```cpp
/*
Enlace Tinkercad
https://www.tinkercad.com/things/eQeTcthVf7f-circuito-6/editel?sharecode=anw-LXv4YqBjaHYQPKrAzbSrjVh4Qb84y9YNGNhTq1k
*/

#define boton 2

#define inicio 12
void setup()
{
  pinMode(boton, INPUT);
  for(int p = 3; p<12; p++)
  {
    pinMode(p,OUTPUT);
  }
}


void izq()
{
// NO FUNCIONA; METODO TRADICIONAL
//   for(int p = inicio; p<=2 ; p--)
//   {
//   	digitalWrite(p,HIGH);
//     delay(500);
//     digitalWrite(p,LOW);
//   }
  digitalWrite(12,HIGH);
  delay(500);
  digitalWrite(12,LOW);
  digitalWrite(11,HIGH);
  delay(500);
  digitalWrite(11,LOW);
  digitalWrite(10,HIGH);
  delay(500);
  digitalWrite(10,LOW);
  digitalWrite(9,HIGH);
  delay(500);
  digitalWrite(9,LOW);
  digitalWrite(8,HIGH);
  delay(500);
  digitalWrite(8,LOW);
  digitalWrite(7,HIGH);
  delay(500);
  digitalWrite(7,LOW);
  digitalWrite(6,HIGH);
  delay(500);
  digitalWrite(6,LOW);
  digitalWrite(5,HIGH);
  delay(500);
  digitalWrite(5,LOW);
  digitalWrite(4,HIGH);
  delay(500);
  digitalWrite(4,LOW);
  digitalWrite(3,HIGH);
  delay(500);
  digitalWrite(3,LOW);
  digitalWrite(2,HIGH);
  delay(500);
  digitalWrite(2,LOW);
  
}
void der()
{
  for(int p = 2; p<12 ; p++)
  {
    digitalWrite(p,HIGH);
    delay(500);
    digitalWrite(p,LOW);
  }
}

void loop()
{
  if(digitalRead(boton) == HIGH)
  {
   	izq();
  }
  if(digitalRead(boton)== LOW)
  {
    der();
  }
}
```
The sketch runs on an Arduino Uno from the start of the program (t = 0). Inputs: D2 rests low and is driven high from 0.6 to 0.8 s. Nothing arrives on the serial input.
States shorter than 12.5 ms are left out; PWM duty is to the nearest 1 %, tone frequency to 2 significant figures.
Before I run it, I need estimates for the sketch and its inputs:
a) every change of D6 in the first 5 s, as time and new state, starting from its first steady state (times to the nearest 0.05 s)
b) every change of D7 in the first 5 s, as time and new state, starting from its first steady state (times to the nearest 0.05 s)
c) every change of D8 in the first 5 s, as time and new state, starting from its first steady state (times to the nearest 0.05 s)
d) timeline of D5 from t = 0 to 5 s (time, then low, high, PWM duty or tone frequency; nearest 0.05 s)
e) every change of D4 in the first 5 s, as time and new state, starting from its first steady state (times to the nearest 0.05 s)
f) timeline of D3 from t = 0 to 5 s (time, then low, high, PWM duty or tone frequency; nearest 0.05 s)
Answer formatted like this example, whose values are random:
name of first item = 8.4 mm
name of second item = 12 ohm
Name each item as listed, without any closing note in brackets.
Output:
every change of D6 in the first 5 s, as time and new state, starting from its first steady state = 0 s low; 2 s high; 2.5 s low
every change of D7 in the first 5 s, as time and new state, starting from its first steady state = 0 s low; 2.5 s high; 3 s low
every change of D8 in the first 5 s, as time and new state, starting from its first steady state = 0 s low; 3 s high; 3.5 s low
timeline of D5 from t = 0 to 5 s = 0 s low; 1.5 s high; 2 s low
every change of D4 in the first 5 s, as time and new state, starting from its first steady state = 0 s low; 1 s high; 1.5 s low
timeline of D3 from t = 0 to 5 s = 0 s low; 0.5 s high; 1 s low
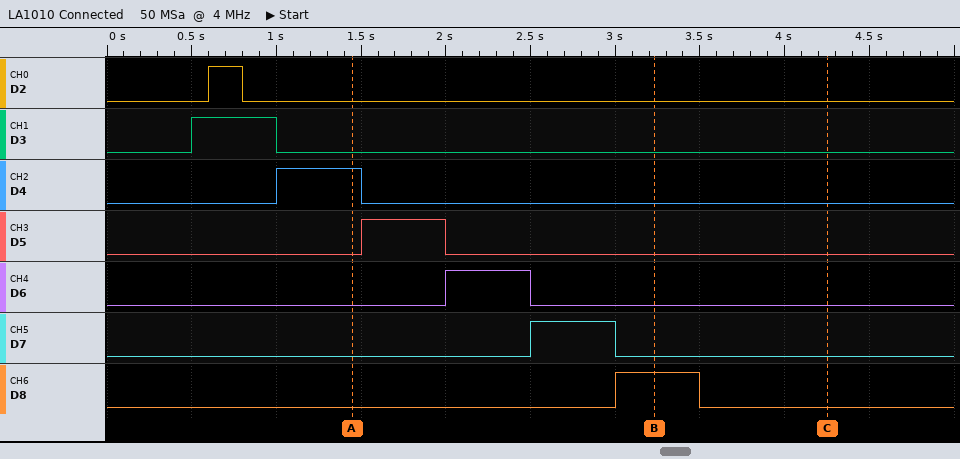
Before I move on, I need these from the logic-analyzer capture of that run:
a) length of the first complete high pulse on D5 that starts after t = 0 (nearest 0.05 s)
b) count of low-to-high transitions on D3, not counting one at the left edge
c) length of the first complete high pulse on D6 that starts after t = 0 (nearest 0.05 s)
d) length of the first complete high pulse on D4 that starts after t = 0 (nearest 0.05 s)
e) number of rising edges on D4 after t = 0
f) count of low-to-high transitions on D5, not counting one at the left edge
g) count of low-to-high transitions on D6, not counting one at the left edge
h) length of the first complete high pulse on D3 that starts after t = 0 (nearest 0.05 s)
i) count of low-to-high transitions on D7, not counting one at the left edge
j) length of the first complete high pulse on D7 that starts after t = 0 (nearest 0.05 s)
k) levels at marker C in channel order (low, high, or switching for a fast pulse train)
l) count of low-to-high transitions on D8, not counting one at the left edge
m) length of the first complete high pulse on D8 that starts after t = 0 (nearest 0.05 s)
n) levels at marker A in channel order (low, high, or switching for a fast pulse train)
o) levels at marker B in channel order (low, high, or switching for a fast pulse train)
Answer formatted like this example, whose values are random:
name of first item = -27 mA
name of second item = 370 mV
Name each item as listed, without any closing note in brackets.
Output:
length of the first complete high pulse on D5 that starts after t = 0 = 0.50 s
count of low-to-high transitions on D3, not counting one at the left edge = 1
length of the first complete high pulse on D6 that starts after t = 0 = 0.50 s
length of the first complete high pulse on D4 that starts after t = 0 = 0.50 s
number of rising edges on D4 after t = 0 = 1
count of low-to-high transitions on D5, not counting one at the left edge = 1
count of low-to-high transitions on D6, not counting one at the left edge = 1
length of the first complete high pulse on D3 that starts after t = 0 = 0.50 s
count of low-to-high transitions on D7, not counting one at the left edge = 1
length of the first complete high pulse on D7 that starts after t = 0 = 0.50 s
levels at marker C in channel order = D2 low, D3 low, D4 low, D5 low, D6 low, D7 low, D8 low
count of low-to-high transitions on D8, not counting one at the left edge = 1
length of the first complete high pulse on D8 that starts after t = 0 = 0.50 s
levels at marker A in channel order = D2 low, D3 low, D4 high, D5 low, D6 low, D7 low, D8 low
levels at marker B in channel order = D2 low, D3 low, D4 low, D5 low, D6 low, D7 low, D8 high
